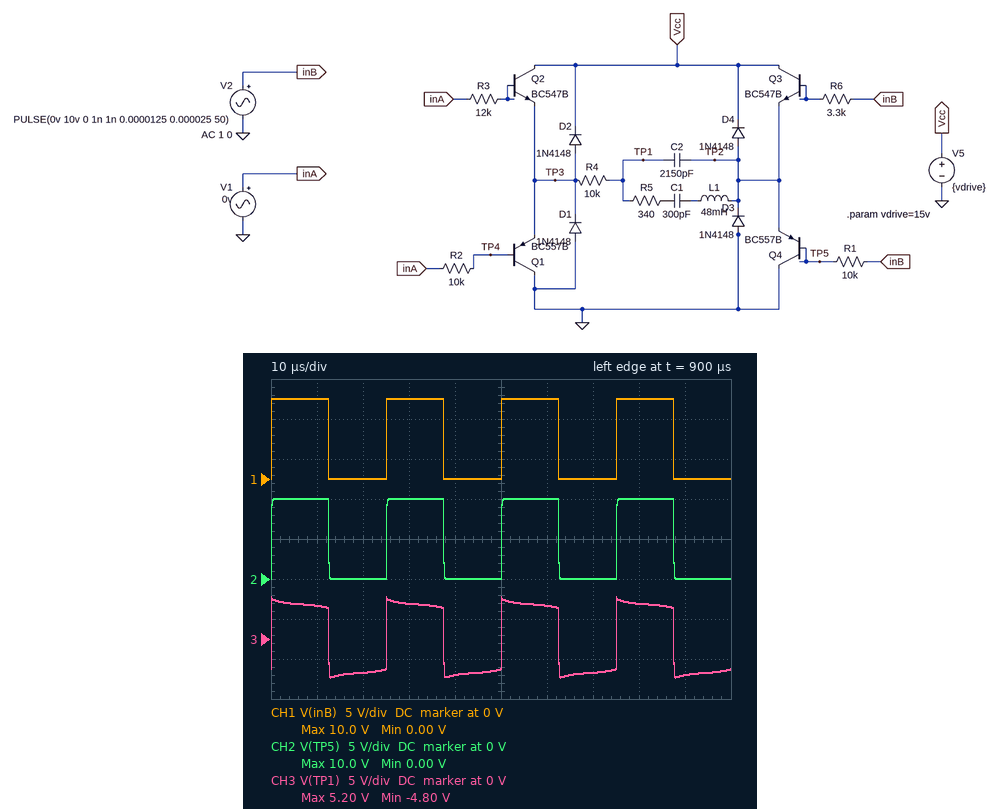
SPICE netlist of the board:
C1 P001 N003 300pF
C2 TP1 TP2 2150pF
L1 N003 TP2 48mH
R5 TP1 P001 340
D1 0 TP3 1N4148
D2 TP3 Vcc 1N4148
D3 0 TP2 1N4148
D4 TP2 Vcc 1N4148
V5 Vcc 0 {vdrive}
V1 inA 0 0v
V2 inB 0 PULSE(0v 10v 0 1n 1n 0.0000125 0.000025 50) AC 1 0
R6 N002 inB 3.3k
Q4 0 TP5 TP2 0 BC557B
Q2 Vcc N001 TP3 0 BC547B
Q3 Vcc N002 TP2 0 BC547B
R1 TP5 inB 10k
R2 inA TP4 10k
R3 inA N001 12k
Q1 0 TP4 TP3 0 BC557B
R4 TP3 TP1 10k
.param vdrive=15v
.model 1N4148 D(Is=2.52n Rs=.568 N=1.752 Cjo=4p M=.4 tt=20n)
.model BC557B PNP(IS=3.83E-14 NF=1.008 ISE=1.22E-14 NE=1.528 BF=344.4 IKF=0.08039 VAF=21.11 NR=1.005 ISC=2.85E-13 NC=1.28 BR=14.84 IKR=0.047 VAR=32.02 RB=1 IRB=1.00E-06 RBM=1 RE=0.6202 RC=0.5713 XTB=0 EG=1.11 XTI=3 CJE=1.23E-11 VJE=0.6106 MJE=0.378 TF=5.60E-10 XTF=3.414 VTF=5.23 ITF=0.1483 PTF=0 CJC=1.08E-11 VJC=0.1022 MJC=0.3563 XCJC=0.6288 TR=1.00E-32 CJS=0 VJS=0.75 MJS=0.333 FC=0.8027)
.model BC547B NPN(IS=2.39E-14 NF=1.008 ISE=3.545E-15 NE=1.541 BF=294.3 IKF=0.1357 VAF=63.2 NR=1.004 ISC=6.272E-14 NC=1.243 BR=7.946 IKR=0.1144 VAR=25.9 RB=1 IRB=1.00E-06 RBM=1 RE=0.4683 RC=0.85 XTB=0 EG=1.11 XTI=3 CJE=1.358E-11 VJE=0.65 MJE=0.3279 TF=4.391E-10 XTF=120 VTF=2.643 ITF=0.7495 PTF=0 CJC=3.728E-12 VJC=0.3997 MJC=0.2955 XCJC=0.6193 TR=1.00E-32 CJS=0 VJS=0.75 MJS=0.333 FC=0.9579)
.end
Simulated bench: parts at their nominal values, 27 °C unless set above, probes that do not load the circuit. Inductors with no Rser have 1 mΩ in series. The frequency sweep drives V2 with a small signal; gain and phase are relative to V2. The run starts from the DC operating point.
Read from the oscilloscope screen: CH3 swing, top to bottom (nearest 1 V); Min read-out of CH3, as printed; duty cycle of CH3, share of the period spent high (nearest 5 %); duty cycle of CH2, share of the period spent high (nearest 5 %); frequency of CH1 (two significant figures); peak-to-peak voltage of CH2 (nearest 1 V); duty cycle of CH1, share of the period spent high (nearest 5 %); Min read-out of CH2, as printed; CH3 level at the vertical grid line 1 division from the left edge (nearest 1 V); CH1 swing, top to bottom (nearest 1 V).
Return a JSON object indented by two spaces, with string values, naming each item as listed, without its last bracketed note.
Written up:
{
  "CH3 swing, top to bottom": "10 V",
  "Min read-out of CH3, as printed": "-4.80 V",
  "duty cycle of CH3, share of the period spent high": "50 %",
  "duty cycle of CH2, share of the period spent high": "50 %",
  "frequency of CH1": "40 kHz",
  "peak-to-peak voltage of CH2": "10 V",
  "duty cycle of CH1, share of the period spent high": "50 %",
  "Min read-out of CH2, as printed": "0.00 V",
  "CH3 level at the vertical grid line 1 division from the left edge": "4 V",
  "CH1 swing, top to bottom": "10 V"
}
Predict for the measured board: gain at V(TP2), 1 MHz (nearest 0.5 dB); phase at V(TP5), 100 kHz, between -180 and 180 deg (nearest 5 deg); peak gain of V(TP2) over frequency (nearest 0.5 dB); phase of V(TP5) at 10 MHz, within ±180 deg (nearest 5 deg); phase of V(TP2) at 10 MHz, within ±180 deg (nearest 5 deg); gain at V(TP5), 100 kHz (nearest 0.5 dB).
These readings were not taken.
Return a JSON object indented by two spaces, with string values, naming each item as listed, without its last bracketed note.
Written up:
{
  "gain at V(TP2), 1 MHz": "-5.5 dB",
  "phase at V(TP5), 100 kHz, between -180 and 180 deg": "-5 deg",
  "peak gain of V(TP2) over frequency": "-5.5 dB",
  "phase of V(TP5) at 10 MHz, within ±180 deg": "-55 deg",
  "phase of V(TP2) at 10 MHz, within ±180 deg": "-50 deg",
  "gain at V(TP5), 100 kHz": "0 dB"
}
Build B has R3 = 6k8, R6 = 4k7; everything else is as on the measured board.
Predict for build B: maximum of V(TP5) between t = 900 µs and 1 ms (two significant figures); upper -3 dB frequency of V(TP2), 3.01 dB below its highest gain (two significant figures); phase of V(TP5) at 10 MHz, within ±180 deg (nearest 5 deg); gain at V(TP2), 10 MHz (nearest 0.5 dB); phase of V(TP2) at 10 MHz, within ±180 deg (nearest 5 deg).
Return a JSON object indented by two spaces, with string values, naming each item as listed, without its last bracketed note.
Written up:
{
  "maximum of V(TP5) between t = 900 µs and 1 ms": "10 V",
  "upper -3 dB frequency of V(TP2), 3.01 dB below its highest gain": "6.2 MHz",
  "phase of V(TP5) at 10 MHz, within ±180 deg": "-65 deg",
  "gain at V(TP2), 10 MHz": "-11.0 dB",
  "phase of V(TP2) at 10 MHz, within ±180 deg": "-60 deg"
}
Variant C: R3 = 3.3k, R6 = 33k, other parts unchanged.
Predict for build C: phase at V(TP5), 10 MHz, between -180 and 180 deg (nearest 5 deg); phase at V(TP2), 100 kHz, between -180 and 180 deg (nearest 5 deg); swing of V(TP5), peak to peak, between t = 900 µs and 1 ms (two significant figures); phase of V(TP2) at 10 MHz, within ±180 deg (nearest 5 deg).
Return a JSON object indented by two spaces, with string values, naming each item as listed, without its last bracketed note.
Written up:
{
  "phase at V(TP5), 10 MHz, between -180 and 180 deg": "-80 deg",
  "phase at V(TP2), 100 kHz, between -180 and 180 deg": "0 deg",
  "swing of V(TP5), peak to peak, between t = 900 µs and 1 ms": "11 V",
  "phase of V(TP2) at 10 MHz, within ±180 deg": "-75 deg"
}
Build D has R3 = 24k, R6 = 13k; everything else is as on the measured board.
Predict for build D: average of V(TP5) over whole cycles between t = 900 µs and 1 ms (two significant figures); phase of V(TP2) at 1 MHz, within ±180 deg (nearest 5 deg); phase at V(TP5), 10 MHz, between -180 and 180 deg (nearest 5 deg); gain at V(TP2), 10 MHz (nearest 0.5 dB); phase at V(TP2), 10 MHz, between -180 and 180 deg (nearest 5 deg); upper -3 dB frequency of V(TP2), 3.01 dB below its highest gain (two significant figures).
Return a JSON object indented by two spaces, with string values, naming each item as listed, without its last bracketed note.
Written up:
{
  "average of V(TP5) over whole cycles between t = 900 µs and 1 ms": "5.0 V",
  "phase of V(TP2) at 1 MHz, within ±180 deg": "-15 deg",
  "phase at V(TP5), 10 MHz, between -180 and 180 deg": "-75 deg",
  "gain at V(TP2), 10 MHz": "-16.0 dB",
  "phase at V(TP2), 10 MHz, between -180 and 180 deg": "-70 deg",
  "upper -3 dB frequency of V(TP2), 3.01 dB below its highest gain": "2.9 MHz"
}
